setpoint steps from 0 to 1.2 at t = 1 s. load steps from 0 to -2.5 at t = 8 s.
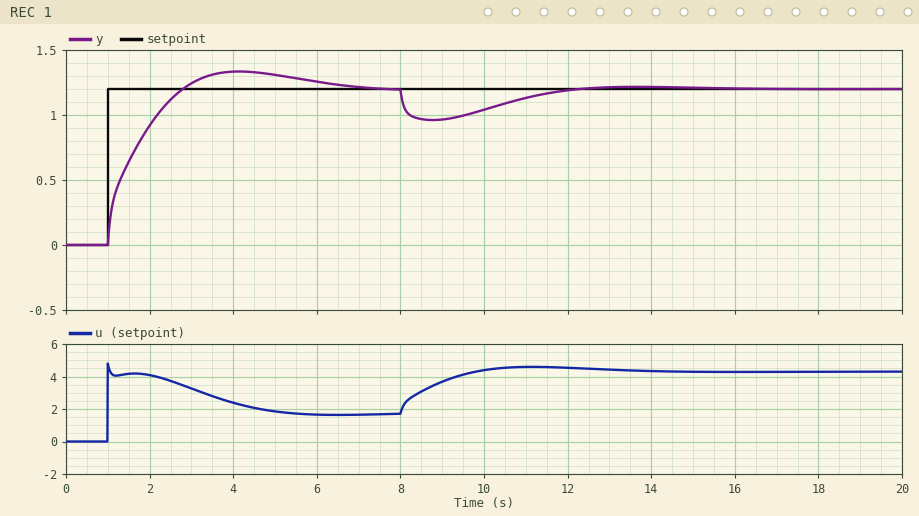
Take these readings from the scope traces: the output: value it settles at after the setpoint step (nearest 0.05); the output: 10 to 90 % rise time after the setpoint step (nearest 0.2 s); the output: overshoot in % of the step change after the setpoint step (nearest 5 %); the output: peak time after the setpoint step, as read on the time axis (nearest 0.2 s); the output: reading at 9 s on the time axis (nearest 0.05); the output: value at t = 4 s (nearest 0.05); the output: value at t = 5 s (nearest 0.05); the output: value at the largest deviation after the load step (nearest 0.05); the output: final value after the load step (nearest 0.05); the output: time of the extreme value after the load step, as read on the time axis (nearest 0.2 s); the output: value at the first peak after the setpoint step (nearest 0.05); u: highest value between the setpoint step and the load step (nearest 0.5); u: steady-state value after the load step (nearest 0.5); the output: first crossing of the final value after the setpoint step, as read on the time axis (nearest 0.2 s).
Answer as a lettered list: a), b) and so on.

a) 1.20
b) 1.4 s
c) 10 %
d) 4.2 s
e) 0.95
f) 1.35
g) 1.30
h) 0.95
i) 1.20
j) 8.8 s
k) 1.35
l) 5.0
m) 4.5
n) 2.8 s
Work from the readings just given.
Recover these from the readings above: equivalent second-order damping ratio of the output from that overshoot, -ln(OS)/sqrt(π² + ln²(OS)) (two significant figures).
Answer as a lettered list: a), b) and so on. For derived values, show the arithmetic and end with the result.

a) ln(0.1) = -2.303; 2.303 / sqrt(9.870 + 5.302) = 0.59
